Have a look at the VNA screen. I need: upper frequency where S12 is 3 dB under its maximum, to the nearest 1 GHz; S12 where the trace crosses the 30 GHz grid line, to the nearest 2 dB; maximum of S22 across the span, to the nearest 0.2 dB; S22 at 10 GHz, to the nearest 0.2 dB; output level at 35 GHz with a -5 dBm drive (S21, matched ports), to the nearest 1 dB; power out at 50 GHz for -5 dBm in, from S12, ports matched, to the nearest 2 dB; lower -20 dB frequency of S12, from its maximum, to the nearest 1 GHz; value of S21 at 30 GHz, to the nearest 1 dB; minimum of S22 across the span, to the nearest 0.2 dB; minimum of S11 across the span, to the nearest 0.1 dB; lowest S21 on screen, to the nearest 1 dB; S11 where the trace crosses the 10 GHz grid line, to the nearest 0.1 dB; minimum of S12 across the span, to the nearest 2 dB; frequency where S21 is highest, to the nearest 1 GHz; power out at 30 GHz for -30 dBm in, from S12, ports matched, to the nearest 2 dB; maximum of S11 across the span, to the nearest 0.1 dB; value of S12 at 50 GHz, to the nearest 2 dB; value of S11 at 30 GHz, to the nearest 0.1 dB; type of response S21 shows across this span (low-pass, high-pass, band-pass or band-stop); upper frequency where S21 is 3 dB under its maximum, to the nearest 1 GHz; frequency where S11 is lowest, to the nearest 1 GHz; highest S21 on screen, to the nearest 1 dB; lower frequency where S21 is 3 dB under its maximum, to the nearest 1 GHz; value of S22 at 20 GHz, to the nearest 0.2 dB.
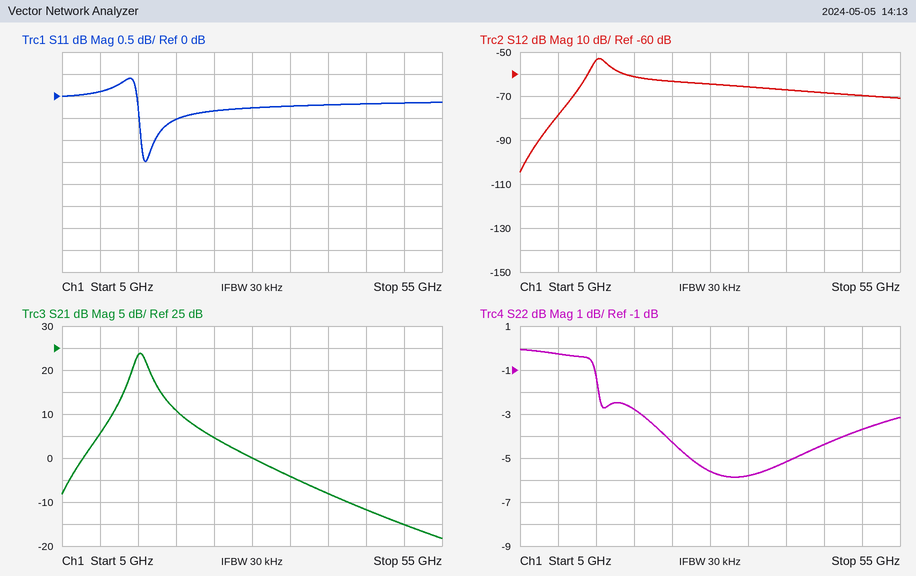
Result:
17 GHz
-64 dB
0.0 dB
-0.2 dB
-9 dBm
-74 dBm
11 GHz
0 dB
-5.8 dB
-1.5 dB
-18 dB
0.1 dB
-104 dB
15 GHz
-94 dBm
0.4 dB
-70 dB
-0.3 dB
band-pass
16 GHz
16 GHz
24 dB
14 GHz
-2.8 dB
